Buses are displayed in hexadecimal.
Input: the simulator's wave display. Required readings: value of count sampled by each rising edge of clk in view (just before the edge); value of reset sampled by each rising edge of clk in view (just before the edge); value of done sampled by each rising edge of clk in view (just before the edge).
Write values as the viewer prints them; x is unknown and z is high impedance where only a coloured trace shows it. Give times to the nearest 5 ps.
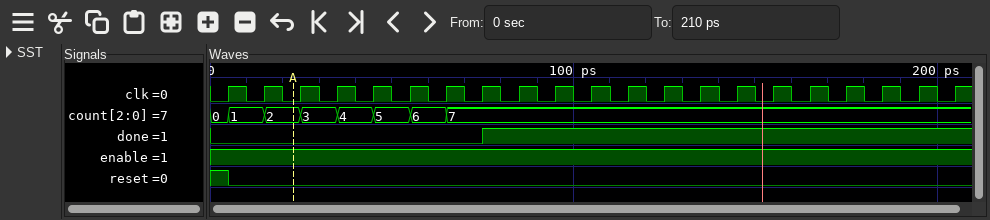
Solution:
0, 1, 2, 3, 4, 5, 6, 7, 7, 7, 7, 7, 7, 7, 7, 7, 7, 7, 7, 7, 7
1 0 0 0 0 0 0 0 0 0 0 0 0 0 0 0 0 0 0 0 0
0 0 0 0 0 0 0 0 1 1 1 1 1 1 1 1 1 1 1 1 1
